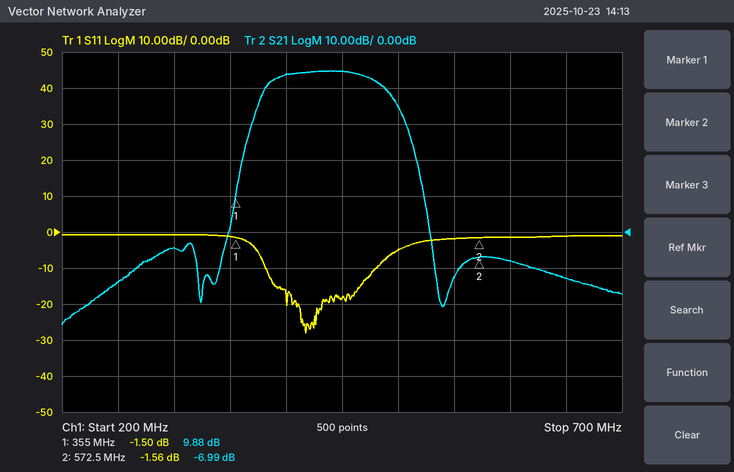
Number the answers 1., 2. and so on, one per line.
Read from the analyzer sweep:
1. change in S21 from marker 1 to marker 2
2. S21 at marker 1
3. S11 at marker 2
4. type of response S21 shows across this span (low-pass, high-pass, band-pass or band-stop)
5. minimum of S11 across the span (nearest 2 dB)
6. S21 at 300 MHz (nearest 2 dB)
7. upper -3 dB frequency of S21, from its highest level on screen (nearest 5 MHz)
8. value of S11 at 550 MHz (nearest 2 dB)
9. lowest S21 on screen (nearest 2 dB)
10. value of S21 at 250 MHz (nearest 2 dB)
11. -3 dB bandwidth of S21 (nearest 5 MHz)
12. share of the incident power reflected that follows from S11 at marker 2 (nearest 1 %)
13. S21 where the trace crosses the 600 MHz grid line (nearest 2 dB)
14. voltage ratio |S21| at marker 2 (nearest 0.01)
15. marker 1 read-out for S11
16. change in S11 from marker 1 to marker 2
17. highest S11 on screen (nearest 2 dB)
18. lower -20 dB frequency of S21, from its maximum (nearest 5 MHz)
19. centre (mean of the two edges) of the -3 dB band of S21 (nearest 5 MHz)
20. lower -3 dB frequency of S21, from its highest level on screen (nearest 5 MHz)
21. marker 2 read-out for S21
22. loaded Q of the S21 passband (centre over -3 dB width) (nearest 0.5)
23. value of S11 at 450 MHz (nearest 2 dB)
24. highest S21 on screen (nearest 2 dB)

1. -16.87 dB
2. 9.88 dB
3. -1.56 dB
4. band-pass
5. -28 dB
6. -4 dB
7. 480 MHz
8. -2 dB
9. -26 dB
10. -14 dB
11. 95 MHz
12. 70 %
13. -8 dB
14. 0.45
15. -1.50 dB
16. -0.06 dB
17. 0 dB
18. 365 MHz
19. 435 MHz
20. 385 MHz
21. -6.99 dB
22. 4.5
23. -18 dB
24. 44 dB
